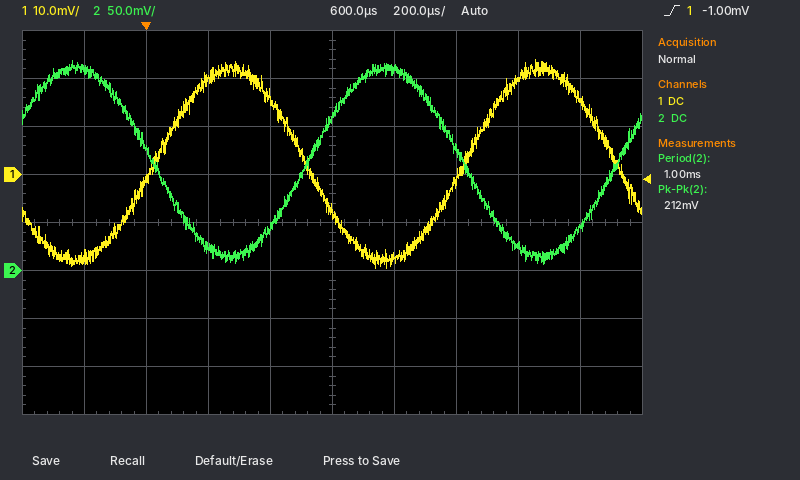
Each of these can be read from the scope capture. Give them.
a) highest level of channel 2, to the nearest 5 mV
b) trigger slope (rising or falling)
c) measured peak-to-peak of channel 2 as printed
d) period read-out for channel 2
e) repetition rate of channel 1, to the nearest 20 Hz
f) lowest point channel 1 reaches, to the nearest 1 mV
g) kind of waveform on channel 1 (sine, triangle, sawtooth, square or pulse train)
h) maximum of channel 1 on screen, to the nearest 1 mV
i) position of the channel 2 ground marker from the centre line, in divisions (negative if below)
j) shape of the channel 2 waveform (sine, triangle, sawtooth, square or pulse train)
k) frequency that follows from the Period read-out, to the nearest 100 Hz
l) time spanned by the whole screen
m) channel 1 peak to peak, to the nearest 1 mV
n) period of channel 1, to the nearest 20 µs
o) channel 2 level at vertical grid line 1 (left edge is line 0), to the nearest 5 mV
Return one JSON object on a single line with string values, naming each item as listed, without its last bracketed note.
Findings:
{"highest level of channel 2, to the nearest 5 mV": "220 mV", "trigger slope": "rising", "measured peak-to-peak of channel 2 as printed": "212 mV", "period read-out for channel 2": "1.00 ms", "repetition rate of channel 1, to the nearest 20 Hz": "1.00 kHz", "lowest point channel 1 reaches, to the nearest 1 mV": "-19 mV", "kind of waveform on channel 1": "sine", "maximum of channel 1 on screen, to the nearest 1 mV": "24 mV", "position of the channel 2 ground marker from the centre line, in divisions": "-1.0 div", "shape of the channel 2 waveform": "sine", "frequency that follows from the Period read-out, to the nearest 100 Hz": "1.0 kHz", "time spanned by the whole screen": "2 ms", "channel 1 peak to peak, to the nearest 1 mV": "43 mV", "period of channel 1, to the nearest 20 µs": "1.00 ms", "channel 2 level at vertical grid line 1 (left edge is line 0), to the nearest 5 mV": "210 mV"}
